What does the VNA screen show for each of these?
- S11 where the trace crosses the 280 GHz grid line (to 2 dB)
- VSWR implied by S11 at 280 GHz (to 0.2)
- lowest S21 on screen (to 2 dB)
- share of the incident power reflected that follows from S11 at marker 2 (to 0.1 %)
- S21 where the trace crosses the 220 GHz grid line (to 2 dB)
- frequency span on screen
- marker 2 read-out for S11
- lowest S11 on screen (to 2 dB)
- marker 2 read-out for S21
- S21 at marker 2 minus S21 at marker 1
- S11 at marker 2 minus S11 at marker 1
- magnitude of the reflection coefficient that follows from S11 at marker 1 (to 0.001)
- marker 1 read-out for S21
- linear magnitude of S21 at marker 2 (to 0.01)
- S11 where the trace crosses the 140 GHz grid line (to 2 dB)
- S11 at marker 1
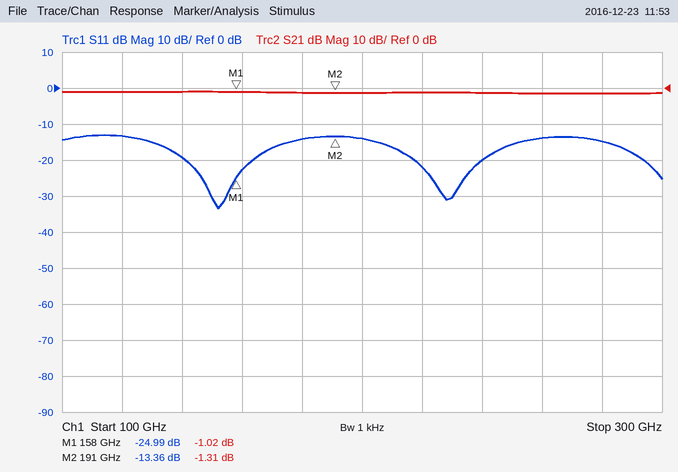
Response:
-14 dB
1.4
-2 dB
4.6 %
-2 dB
200 GHz
-13.36 dB
-34 dB
-1.31 dB
-0.29 dB
11.63 dB
0.056
-1.02 dB
0.86
-20 dB
-24.99 dB
